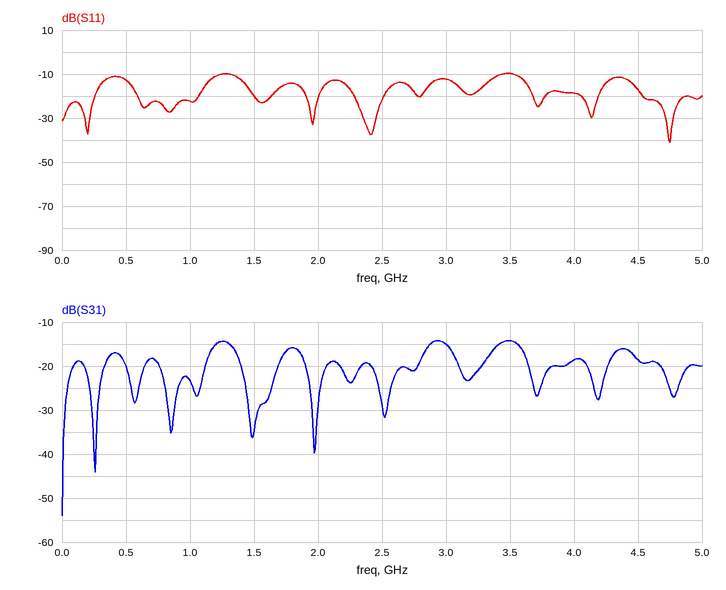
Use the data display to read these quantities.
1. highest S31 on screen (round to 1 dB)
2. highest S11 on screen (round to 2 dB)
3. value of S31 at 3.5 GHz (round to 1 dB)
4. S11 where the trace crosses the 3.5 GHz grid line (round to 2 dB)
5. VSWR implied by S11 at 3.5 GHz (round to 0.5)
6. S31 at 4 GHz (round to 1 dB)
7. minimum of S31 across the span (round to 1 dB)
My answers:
-14 dB
-10 dB
-14 dB
-10 dB
2.0
-19 dB
-54 dB
